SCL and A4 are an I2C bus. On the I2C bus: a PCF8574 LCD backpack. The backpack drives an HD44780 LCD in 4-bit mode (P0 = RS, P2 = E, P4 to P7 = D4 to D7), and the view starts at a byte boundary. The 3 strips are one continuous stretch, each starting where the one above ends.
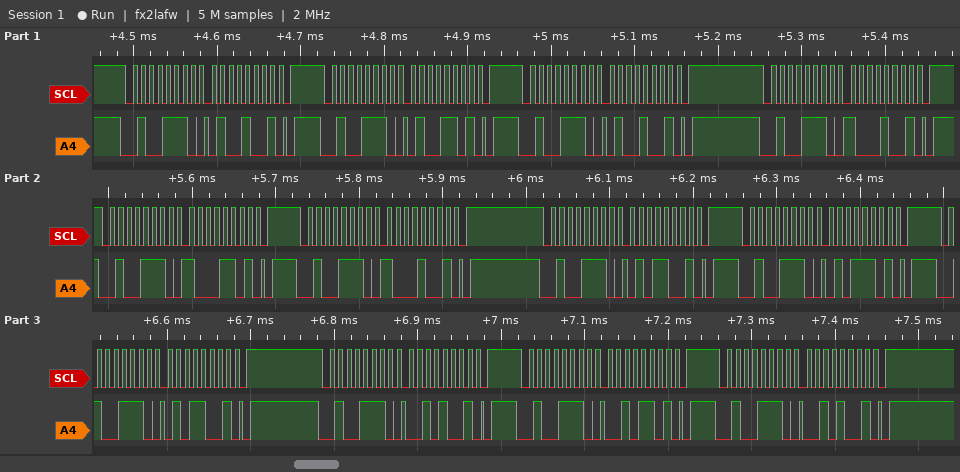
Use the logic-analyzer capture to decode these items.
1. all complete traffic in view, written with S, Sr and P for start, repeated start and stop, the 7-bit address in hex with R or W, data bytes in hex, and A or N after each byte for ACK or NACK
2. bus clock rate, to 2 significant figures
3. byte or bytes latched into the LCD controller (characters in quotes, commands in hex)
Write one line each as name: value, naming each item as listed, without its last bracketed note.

all complete traffic in view, written with S, Sr and P for start, repeated start and stop, the 7-bit address in hex with R or W, data bytes in hex, and A or N after each byte for ACK or NACK: S 27W A 49 A P S 27W A 4D A P S 27W A 49 A P S 27W A 89 A P S 27W A 8D A P S 27W A 89 A P S 27W A 59 A P S 27W A 5D A P S 27W A 59 A P S 27W A 29 A P S 27W A 2D A P S 27W A 29 A P
bus clock rate, to 2 significant figures: 100 kHz
byte or bytes latched into the LCD controller: 'H' 'R'
